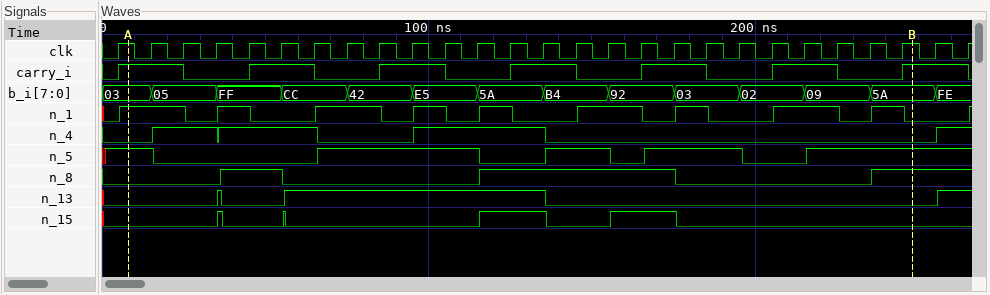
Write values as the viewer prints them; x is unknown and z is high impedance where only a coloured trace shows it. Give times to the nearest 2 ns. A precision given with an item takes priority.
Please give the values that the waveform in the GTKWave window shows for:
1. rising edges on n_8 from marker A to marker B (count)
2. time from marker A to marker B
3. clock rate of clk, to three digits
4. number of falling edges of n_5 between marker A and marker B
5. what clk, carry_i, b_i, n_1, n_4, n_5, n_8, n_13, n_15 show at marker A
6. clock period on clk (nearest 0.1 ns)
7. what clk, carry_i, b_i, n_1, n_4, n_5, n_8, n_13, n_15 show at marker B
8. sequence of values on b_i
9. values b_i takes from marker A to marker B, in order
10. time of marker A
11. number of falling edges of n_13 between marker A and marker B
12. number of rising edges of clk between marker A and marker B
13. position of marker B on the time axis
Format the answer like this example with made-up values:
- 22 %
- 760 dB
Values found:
- 3
- 240 ns
- 100 MHz
- 4
- clk=1, carry_i=1, b_i=03, n_1=1, n_4=0, n_5=1, n_8=0, n_13=0, n_15=0
- 10 ns
- clk=1, carry_i=1, b_i=5A, n_1=0, n_4=0, n_5=1, n_8=1, n_13=0, n_15=0
- 03, 05, FF, CC, 42, E5, 5A, B4, 92, 03, 02, 09, 5A, FE
- 03, 05, FF, CC, 42, E5, 5A, B4, 92, 03, 02, 09, 5A
- 8 ns
- 2
- 24
- 248 ns
